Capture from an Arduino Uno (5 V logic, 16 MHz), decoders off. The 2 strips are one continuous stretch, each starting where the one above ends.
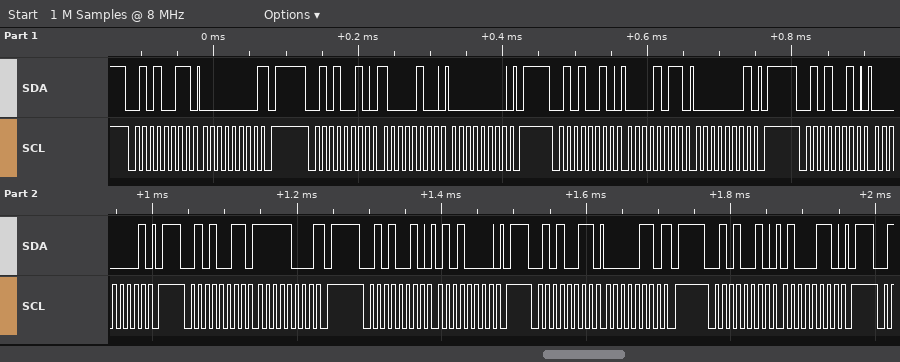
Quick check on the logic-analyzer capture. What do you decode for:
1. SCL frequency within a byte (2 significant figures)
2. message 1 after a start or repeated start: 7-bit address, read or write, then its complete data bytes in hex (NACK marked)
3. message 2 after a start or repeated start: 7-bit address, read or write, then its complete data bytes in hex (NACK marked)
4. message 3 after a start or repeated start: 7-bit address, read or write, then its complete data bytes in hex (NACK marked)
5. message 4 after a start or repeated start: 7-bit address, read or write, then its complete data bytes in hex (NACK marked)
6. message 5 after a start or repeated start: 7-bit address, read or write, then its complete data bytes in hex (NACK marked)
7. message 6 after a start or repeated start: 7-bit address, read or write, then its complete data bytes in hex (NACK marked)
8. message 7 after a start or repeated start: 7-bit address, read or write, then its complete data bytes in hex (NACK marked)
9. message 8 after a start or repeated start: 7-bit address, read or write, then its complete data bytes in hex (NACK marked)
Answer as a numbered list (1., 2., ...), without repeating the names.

1. 100 kHz
2. 0x29 read: 00 NACK
3. 0x29 write: 84 00
4. 0x29 write: 0B 01
5. 0x29 write: 01
6. 0x29 read: F8 NACK
7. 0x29 write: 50
8. 0x29 read: 06 NACK
9. 0x29 write: 46
